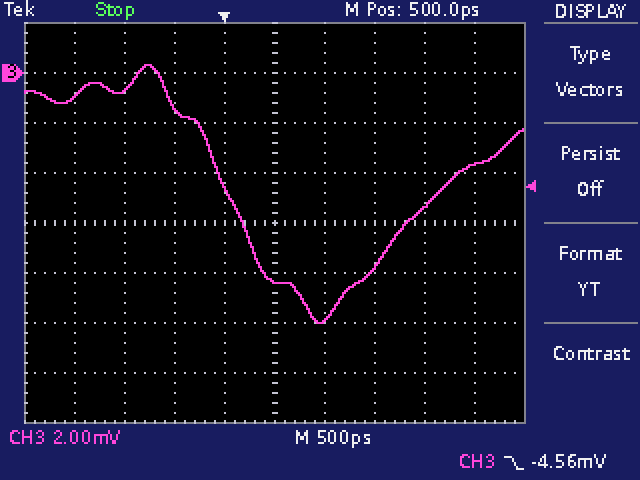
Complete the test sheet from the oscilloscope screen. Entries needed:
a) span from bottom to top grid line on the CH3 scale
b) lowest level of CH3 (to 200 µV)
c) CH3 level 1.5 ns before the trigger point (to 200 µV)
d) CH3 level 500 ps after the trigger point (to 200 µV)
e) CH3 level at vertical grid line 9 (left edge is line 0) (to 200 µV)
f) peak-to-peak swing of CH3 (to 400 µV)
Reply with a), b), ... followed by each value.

a) 16 mV
b) -10.0 mV
c) -1.0 mV
d) -8.4 mV
e) -3.6 mV
f) 10.4 mV
